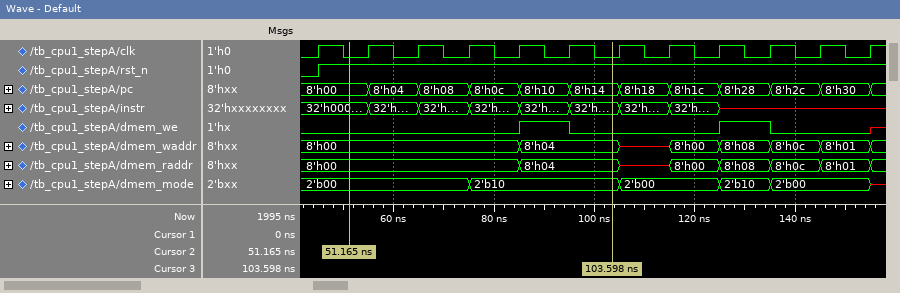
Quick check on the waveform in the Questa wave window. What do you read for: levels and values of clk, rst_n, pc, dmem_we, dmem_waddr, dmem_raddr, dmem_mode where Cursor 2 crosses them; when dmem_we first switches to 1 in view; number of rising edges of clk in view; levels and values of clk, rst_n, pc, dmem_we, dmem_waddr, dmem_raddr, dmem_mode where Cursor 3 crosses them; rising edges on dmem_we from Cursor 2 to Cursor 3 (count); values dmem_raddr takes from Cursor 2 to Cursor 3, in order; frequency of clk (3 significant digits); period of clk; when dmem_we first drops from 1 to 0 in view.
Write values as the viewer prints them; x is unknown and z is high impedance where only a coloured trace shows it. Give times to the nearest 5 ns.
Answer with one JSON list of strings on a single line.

["clk=0, rst_n=1, pc=8'h00, dmem_we=0, dmem_waddr=8'h00, dmem_raddr=8'h00, dmem_mode=2'b00", "85 ns", "12", "clk=0, rst_n=1, pc=8'h14, dmem_we=0, dmem_waddr=8'h04, dmem_raddr=8'h04, dmem_mode=2'b10", "1", "8'h00, 8'h04", "100 MHz", "10 ns", "95 ns"]
